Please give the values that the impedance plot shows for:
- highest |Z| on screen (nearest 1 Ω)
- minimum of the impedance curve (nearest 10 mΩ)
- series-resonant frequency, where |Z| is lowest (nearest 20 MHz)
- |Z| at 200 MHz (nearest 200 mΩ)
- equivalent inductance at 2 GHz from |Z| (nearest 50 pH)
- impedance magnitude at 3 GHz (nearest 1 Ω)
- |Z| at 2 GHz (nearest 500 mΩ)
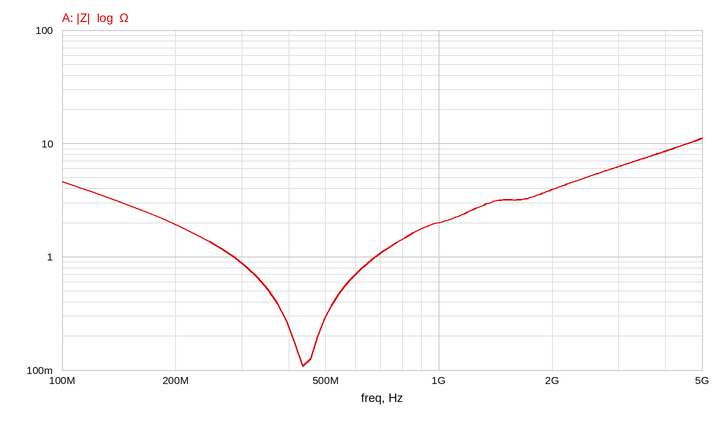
11 Ω
110 mΩ
440 MHz
2.0 Ω
300 pH
6 Ω
4.0 Ω
